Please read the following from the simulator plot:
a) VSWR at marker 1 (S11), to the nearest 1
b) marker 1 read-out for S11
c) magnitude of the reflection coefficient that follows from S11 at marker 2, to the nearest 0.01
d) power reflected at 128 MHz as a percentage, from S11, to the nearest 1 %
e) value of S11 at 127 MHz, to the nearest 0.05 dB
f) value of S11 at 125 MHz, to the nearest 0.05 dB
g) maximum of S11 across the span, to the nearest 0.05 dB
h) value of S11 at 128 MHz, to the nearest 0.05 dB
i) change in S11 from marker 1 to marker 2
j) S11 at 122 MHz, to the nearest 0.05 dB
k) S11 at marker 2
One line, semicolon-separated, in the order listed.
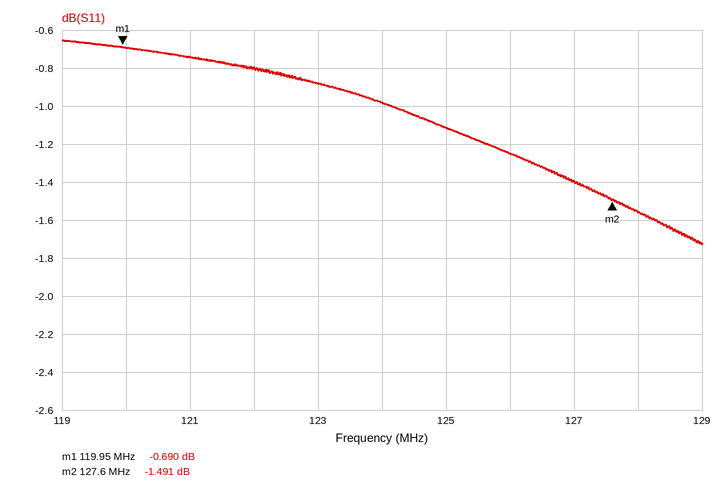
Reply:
25; -0.690 dB; 0.84; 70 %; -1.40 dB; -1.10 dB; -0.65 dB; -1.55 dB; -0.801 dB; -0.80 dB; -1.491 dB
